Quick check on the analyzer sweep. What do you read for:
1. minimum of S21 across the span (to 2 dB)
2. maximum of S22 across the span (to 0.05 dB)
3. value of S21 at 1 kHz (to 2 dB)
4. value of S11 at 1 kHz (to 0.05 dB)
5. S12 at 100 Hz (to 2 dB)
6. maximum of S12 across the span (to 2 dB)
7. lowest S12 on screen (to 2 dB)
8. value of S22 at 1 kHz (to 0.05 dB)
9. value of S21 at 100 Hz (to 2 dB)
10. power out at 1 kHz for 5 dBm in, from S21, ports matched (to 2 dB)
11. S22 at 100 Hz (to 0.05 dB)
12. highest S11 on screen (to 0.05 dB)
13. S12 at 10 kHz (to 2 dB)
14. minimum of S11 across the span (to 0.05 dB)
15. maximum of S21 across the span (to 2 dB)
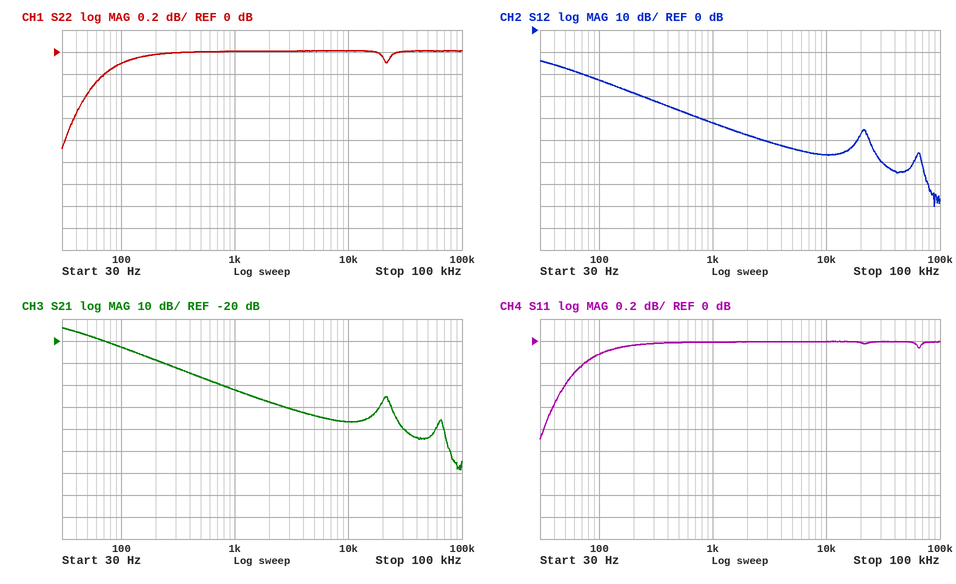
-78 dB
0.00 dB
-42 dB
0.00 dB
-22 dB
-14 dB
-80 dB
0.00 dB
-22 dB
-38 dBm
-0.10 dB
0.00 dB
-56 dB
-0.90 dB
-14 dB
